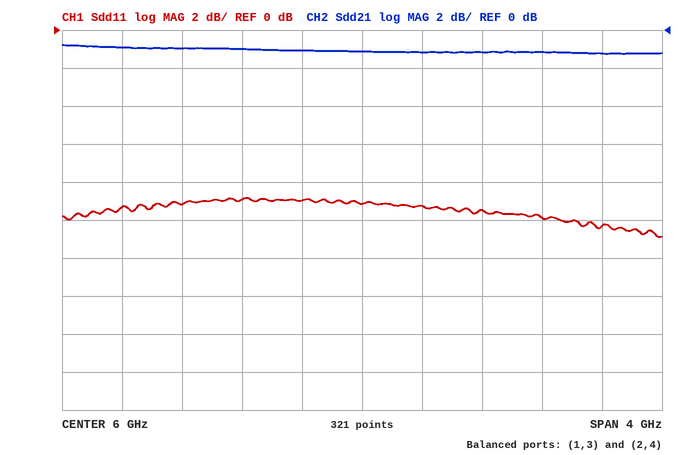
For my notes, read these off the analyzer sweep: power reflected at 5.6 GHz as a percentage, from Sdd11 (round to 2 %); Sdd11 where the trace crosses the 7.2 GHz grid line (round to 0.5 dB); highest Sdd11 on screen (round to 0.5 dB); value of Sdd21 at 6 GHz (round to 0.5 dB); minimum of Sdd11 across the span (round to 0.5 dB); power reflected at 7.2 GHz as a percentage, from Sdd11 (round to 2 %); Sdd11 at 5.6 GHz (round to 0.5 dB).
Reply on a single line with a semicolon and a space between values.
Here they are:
12 %; -10.0 dB; -9.0 dB; -1.0 dB; -11.0 dB; 10 %; -9.0 dB
